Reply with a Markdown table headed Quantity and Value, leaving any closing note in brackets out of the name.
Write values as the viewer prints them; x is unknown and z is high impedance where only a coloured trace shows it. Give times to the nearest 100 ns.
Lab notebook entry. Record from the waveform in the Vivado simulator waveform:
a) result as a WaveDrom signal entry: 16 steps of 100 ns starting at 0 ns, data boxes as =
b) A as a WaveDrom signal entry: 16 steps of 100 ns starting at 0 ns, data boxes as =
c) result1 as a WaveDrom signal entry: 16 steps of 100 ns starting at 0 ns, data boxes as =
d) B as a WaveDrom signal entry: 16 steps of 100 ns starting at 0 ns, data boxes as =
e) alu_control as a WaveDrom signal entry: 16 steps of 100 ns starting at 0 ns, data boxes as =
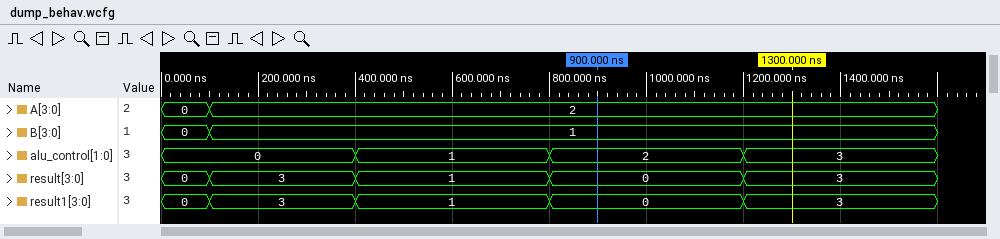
| Quantity | Value |
|---|---|
| result as a WaveDrom signal entry: 16 steps of 100 ns starting at 0 ns, data boxes as = | {name: 'result', wave: '==..=...=...=...', data: '0 3 1 0 3'} |
| A as a WaveDrom signal entry: 16 steps of 100 ns starting at 0 ns, data boxes as = | {name: 'A', wave: '==..............', data: '0 2'} |
| result1 as a WaveDrom signal entry: 16 steps of 100 ns starting at 0 ns, data boxes as = | {name: 'result1', wave: '==..=...=...=...', data: '0 3 1 0 3'} |
| B as a WaveDrom signal entry: 16 steps of 100 ns starting at 0 ns, data boxes as = | {name: 'B', wave: '==..............', data: '0 1'} |
| alu_control as a WaveDrom signal entry: 16 steps of 100 ns starting at 0 ns, data boxes as = | {name: 'alu_control', wave: '=...=...=...=...', data: '0 1 2 3'} |
